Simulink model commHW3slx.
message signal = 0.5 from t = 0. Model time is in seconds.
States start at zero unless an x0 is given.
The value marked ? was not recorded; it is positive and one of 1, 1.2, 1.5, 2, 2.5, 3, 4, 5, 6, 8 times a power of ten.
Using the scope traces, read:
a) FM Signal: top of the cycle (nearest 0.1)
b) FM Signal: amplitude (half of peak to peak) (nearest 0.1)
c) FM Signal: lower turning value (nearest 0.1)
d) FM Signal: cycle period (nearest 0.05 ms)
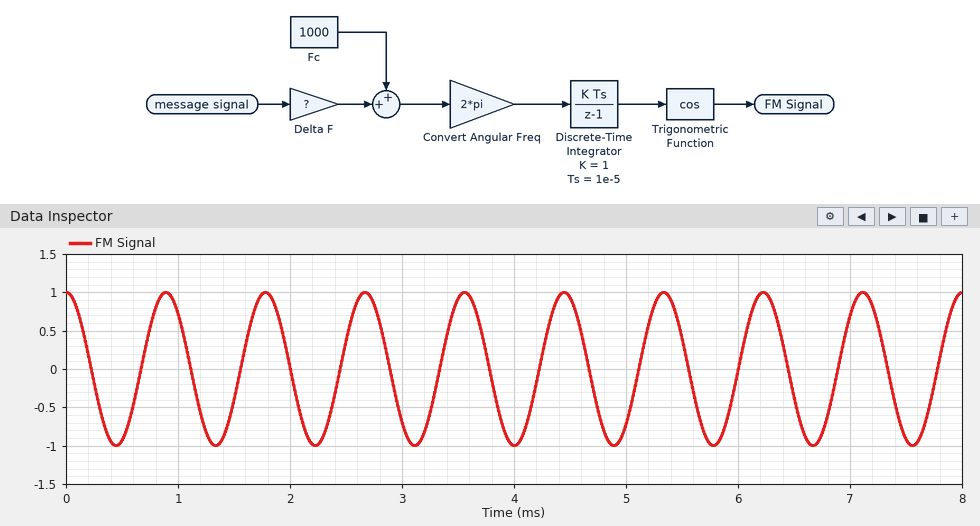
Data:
1.0
1.0
-1.0
0.90 ms
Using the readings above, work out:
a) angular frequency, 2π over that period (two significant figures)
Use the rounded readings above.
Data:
7.0 rad/ms
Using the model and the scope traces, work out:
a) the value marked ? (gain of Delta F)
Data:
250
